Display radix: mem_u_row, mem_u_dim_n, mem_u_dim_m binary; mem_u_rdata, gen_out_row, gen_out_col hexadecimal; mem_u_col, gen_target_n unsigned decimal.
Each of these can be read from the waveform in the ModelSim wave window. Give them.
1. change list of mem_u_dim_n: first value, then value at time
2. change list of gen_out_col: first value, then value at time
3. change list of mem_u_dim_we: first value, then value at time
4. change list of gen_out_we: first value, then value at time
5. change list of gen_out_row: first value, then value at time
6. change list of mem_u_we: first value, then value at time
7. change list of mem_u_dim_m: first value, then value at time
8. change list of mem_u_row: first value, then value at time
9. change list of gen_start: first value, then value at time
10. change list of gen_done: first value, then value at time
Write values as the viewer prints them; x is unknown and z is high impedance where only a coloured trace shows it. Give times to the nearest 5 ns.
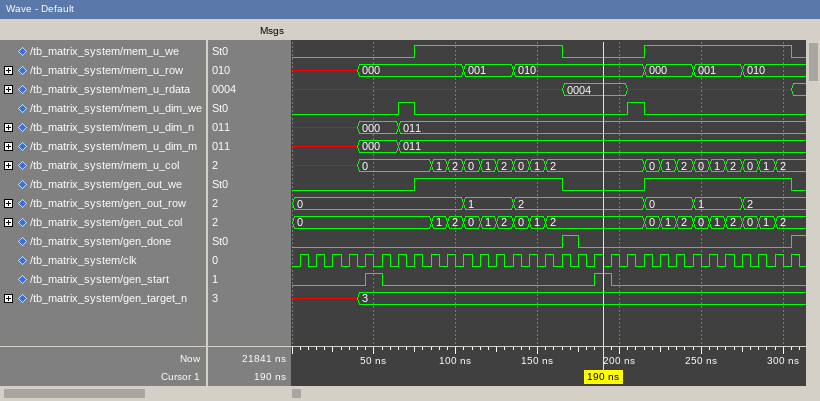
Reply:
x, 000 at 40 ns, 011 at 65 ns
0, 1 at 85 ns, 2 at 95 ns, 0 at 105 ns, 1 at 115 ns, 2 at 125 ns, 0 at 135 ns, 1 at 145 ns, 2 at 155 ns, 0 at 215 ns, 1 at 225 ns, 2 at 235 ns, 0 at 245 ns, 1 at 255 ns, 2 at 265 ns, 0 at 275 ns, 1 at 285 ns, 2 at 295 ns
0, 1 at 65 ns, 0 at 75 ns, 1 at 205 ns, 0 at 215 ns
0, 1 at 75 ns, 0 at 165 ns, 1 at 215 ns, 0 at 305 ns
0, 1 at 105 ns, 2 at 135 ns, 0 at 215 ns, 1 at 245 ns, 2 at 275 ns
0, 1 at 75 ns, 0 at 165 ns, 1 at 215 ns, 0 at 305 ns
x, 000 at 40 ns, 011 at 65 ns
x, 000 at 40 ns, 001 at 105 ns, 010 at 135 ns, 000 at 215 ns, 001 at 245 ns, 010 at 275 ns
0, 1 at 45 ns, 0 at 55 ns, 1 at 185 ns, 0 at 195 ns
0, 1 at 165 ns, 0 at 175 ns, 1 at 305 ns
